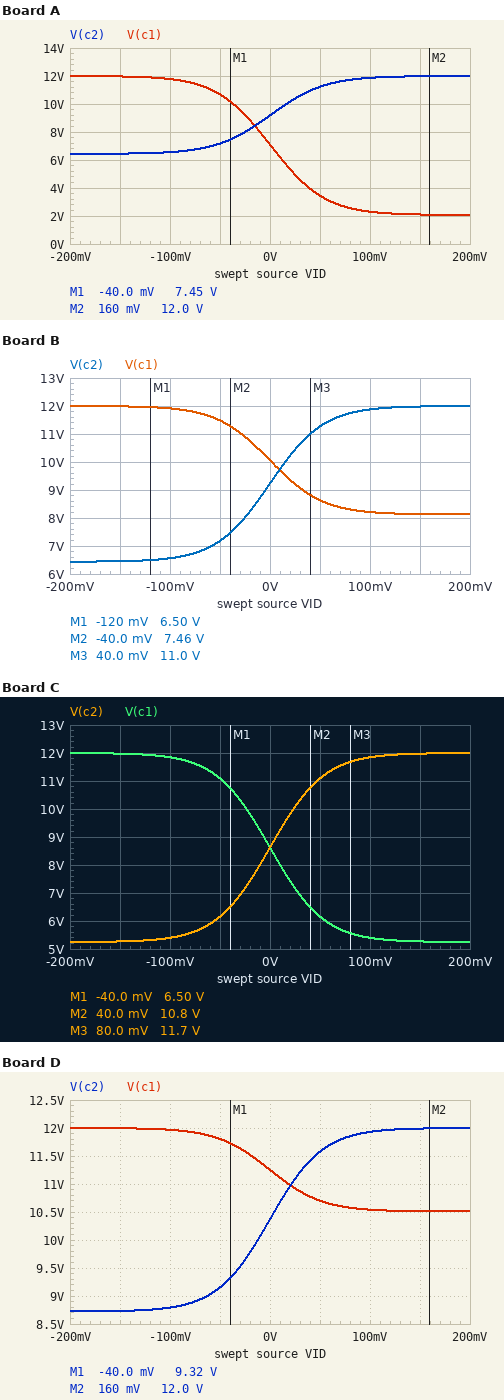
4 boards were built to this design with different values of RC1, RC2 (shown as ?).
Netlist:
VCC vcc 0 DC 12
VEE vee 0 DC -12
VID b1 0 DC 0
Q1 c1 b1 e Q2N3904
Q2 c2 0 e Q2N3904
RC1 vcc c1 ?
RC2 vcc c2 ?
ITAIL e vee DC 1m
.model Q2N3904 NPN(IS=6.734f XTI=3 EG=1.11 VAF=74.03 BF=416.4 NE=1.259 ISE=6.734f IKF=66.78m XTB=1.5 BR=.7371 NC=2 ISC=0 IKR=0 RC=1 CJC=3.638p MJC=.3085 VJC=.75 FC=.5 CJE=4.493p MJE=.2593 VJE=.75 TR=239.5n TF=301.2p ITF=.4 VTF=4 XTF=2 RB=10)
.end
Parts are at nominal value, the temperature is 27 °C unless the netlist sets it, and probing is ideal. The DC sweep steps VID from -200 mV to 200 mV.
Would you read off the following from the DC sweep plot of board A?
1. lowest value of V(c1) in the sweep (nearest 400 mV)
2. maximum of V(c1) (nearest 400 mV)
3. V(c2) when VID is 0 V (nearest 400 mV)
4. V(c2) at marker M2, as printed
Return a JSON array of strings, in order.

["2.0 V", "12.0 V", "9.2 V", "12.0 V"]
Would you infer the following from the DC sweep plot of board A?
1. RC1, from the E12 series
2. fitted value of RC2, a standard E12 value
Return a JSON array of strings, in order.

["10 kΩ", "5.6 kΩ"]
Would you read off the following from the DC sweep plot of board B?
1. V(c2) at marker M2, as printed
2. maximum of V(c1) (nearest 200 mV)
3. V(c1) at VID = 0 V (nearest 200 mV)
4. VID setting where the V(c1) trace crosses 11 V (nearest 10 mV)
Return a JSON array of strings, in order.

["7.46 V", "12.0 V", "10.0 V", "-30 mV"]
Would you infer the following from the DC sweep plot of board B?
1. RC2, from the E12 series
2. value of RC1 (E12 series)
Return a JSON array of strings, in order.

["5.6 kΩ", "3.9 kΩ"]
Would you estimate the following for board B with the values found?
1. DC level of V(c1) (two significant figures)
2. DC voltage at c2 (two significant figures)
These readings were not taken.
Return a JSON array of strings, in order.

["10 V", "9.2 V"]
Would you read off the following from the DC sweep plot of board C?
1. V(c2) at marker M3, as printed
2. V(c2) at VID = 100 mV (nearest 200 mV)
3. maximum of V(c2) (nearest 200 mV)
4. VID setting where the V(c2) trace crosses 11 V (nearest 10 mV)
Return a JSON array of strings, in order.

["11.7 V", "11.8 V", "12.0 V", "50 mV"]
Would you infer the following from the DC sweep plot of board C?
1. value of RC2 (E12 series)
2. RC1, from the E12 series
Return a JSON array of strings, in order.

["6.8 kΩ", "6.8 kΩ"]
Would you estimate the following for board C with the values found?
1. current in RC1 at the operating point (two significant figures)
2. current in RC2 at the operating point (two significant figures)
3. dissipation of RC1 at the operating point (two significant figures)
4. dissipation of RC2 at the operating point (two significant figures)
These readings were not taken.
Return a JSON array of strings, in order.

["500 µA", "500 µA", "1.7 mW", "1.7 mW"]
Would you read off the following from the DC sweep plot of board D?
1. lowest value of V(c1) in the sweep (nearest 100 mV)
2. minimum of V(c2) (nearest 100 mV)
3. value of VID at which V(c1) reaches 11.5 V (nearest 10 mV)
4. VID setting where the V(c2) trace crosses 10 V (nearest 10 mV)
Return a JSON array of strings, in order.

["10.5 V", "8.7 V", "-20 mV", "-10 mV"]
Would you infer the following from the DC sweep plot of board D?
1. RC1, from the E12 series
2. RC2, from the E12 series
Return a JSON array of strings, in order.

["1.5 kΩ", "3.3 kΩ"]
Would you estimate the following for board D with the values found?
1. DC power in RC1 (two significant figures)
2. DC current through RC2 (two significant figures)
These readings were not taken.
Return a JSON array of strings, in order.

["370 µW", "490 µA"]
